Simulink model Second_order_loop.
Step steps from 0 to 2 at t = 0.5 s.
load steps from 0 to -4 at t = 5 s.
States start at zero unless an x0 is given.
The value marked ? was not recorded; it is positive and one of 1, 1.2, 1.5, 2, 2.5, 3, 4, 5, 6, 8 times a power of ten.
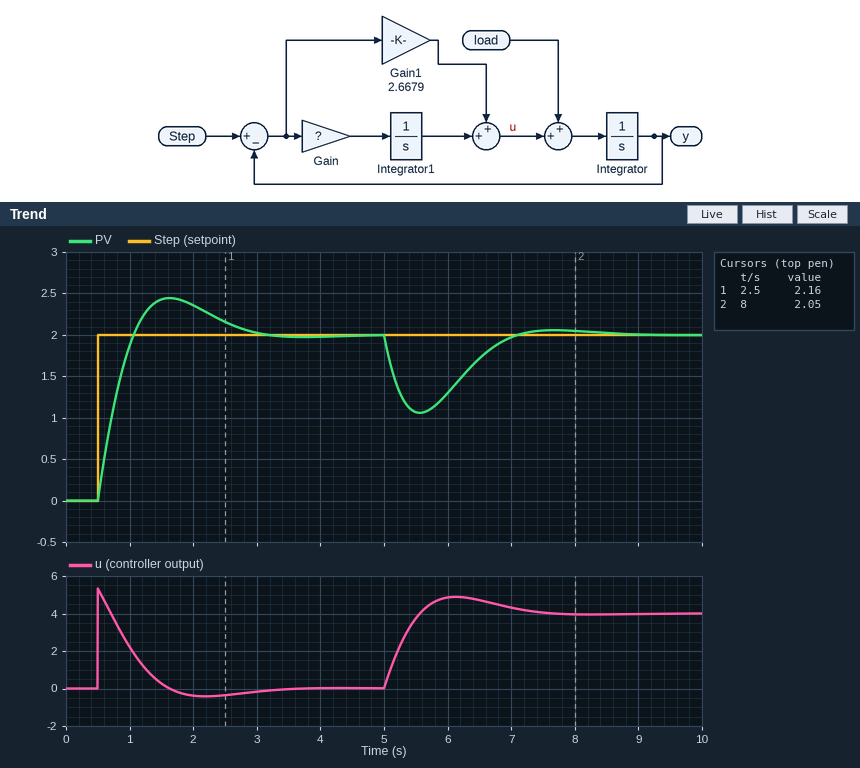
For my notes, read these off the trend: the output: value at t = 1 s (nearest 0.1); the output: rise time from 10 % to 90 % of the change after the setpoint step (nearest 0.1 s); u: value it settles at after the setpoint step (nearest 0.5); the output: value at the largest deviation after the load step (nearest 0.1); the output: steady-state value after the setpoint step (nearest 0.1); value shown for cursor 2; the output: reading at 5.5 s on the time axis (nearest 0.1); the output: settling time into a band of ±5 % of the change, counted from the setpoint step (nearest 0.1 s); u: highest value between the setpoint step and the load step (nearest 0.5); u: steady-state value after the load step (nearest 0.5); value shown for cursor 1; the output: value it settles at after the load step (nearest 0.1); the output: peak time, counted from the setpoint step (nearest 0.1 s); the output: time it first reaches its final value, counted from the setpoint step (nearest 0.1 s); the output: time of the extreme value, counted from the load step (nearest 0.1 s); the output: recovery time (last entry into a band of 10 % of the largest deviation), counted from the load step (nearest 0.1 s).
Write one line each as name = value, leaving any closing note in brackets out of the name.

the output: value at t = 1 s = 1.9
the output: rise time from 10 % to 90 % of the change after the setpoint step = 0.4 s
u: value it settles at after the setpoint step = 0.0
the output: value at the largest deviation after the load step = 1.1
the output: steady-state value after the setpoint step = 2.0
value shown for cursor 2 = 2.05
the output: reading at 5.5 s on the time axis = 1.1
the output: settling time into a band of ±5 % of the change, counted from the setpoint step = 2.2 s
u: highest value between the setpoint step and the load step = 5.5
u: steady-state value after the load step = 4.0
value shown for cursor 1 = 2.16
the output: value it settles at after the load step = 2.0
the output: peak time, counted from the setpoint step = 1.1 s
the output: time it first reaches its final value, counted from the setpoint step = 0.6 s
the output: time of the extreme value, counted from the load step = 0.6 s
the output: recovery time (last entry into a band of 10 % of the largest deviation), counted from the load step = 1.8 s
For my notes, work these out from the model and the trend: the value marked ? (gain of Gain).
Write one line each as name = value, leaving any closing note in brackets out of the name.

the value marked ? = 4
